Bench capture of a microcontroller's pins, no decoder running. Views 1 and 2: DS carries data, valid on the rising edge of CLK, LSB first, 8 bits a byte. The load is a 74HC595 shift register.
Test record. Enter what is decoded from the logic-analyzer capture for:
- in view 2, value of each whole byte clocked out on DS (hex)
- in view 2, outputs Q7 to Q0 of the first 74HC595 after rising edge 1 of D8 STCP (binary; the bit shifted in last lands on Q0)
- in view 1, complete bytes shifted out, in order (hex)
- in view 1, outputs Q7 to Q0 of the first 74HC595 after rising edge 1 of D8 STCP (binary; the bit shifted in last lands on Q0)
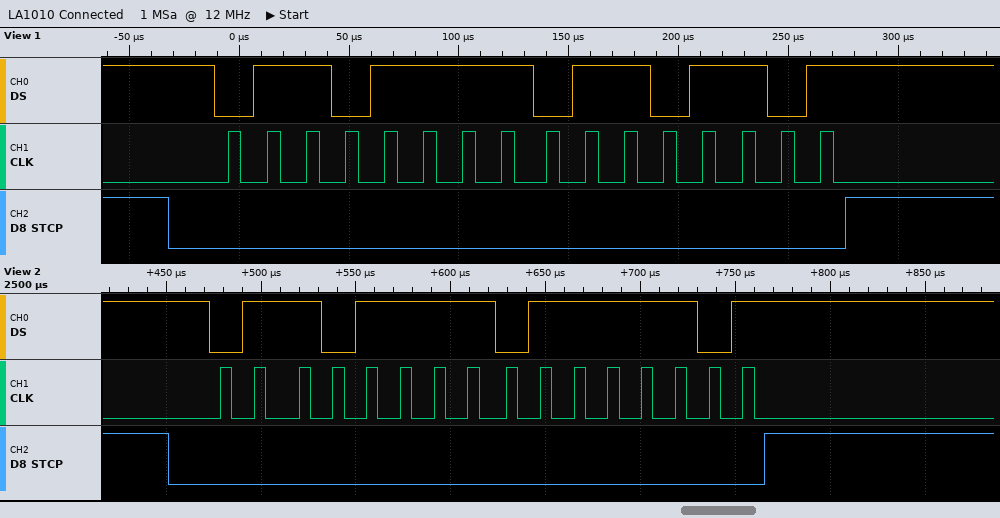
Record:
0xF6 0xBE
01111101
F6 B6
01101101
